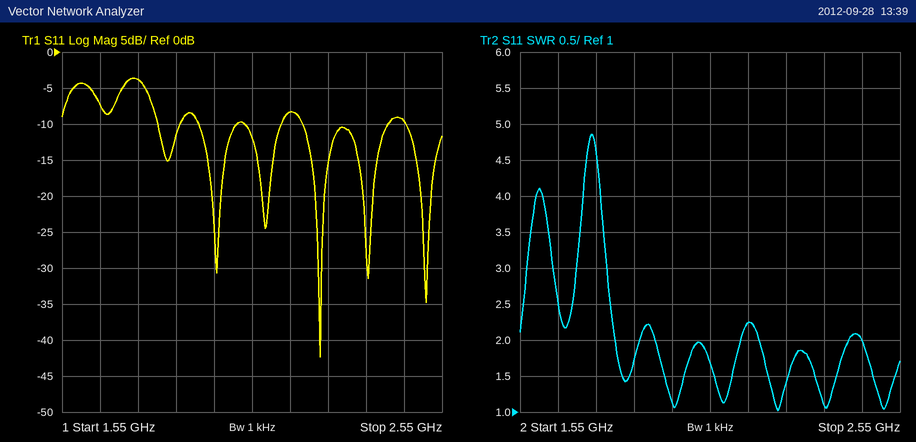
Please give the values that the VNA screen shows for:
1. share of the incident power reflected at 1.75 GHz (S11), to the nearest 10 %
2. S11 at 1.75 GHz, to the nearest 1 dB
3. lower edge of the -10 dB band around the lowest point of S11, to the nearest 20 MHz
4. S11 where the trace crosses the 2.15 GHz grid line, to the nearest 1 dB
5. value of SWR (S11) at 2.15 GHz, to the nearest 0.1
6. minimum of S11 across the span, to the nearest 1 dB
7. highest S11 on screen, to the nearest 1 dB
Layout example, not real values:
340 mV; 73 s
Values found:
40 %; -4 dB; 2.18 GHz; -8 dB; 2.2; -42 dB; -4 dB
